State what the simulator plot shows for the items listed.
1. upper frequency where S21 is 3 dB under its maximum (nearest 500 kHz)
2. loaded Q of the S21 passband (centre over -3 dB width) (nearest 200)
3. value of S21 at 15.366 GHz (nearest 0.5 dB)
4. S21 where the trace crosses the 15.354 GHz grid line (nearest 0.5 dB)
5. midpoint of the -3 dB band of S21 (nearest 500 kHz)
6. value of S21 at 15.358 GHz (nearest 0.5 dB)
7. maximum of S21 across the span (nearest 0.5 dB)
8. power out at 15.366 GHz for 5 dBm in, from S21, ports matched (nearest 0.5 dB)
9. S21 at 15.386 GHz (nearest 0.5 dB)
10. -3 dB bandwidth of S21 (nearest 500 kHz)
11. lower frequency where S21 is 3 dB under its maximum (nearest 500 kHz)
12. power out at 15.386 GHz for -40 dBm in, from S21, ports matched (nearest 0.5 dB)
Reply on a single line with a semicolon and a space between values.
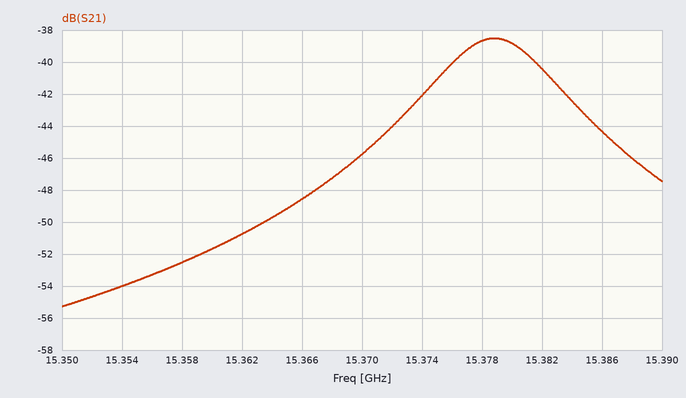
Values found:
15.3830 GHz; 1800; -48.5 dB; -54.0 dB; 15.3790 GHz; -52.5 dB; -38.5 dB; -43.5 dBm; -44.5 dB; 8.5 MHz; 15.3745 GHz; -84.5 dBm
